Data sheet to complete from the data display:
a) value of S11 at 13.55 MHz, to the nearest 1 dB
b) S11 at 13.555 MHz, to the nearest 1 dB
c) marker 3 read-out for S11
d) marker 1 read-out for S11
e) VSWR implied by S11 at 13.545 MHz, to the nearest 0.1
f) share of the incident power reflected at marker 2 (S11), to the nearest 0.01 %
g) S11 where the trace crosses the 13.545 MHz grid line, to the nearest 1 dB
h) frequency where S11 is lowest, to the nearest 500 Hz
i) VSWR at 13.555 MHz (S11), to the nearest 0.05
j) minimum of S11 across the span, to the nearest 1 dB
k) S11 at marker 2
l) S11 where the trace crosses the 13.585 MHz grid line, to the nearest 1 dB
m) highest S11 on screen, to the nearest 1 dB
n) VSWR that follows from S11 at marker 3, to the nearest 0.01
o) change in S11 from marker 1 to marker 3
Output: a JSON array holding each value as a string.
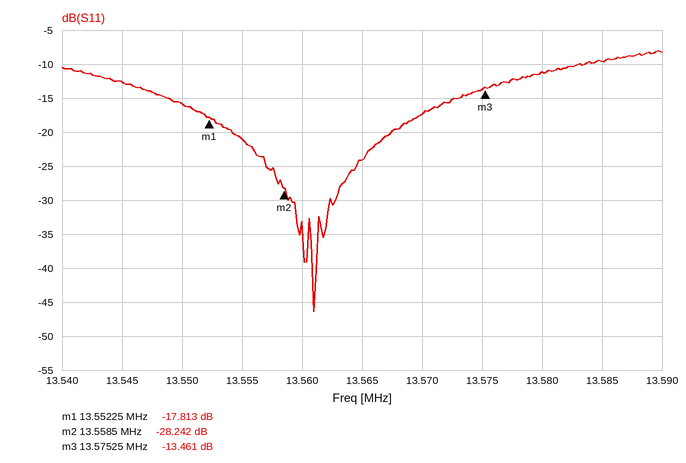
["-16 dB", "-21 dB", "-13.461 dB", "-17.813 dB", "1.6", "0.15 %", "-13 dB", "13.5610 MHz", "1.20", "-46 dB", "-28.242 dB", "-10 dB", "-8 dB", "1.54", "4.352 dB"]
